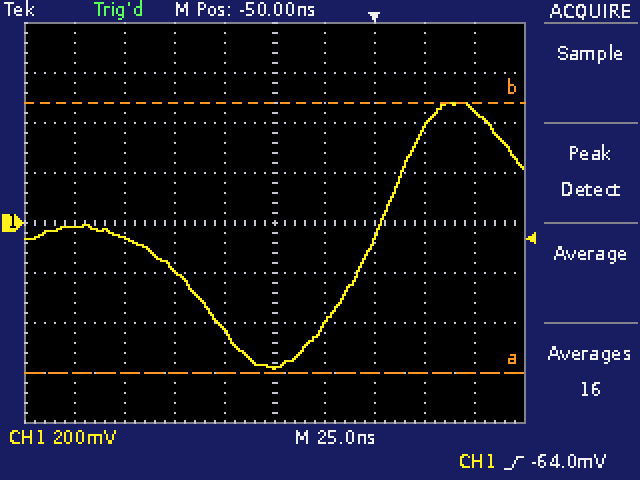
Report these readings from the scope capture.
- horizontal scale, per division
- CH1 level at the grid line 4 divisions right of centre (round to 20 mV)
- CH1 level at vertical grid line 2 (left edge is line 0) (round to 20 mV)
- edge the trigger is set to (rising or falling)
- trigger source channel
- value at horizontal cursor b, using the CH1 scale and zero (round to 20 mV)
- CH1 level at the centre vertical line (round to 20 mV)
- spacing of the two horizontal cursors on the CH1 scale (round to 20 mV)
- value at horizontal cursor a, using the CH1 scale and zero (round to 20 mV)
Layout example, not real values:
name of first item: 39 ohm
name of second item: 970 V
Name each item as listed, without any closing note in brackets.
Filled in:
horizontal scale, per division: 25 ns
CH1 level at the grid line 4 divisions right of centre: 440 mV
CH1 level at vertical grid line 2 (left edge is line 0): -60 mV
edge the trigger is set to: rising
trigger source channel: CH1
value at horizontal cursor b, using the CH1 scale and zero: 480 mV
CH1 level at the centre vertical line: -580 mV
spacing of the two horizontal cursors on the CH1 scale: 1.08 V
value at horizontal cursor a, using the CH1 scale and zero: -600 mV
